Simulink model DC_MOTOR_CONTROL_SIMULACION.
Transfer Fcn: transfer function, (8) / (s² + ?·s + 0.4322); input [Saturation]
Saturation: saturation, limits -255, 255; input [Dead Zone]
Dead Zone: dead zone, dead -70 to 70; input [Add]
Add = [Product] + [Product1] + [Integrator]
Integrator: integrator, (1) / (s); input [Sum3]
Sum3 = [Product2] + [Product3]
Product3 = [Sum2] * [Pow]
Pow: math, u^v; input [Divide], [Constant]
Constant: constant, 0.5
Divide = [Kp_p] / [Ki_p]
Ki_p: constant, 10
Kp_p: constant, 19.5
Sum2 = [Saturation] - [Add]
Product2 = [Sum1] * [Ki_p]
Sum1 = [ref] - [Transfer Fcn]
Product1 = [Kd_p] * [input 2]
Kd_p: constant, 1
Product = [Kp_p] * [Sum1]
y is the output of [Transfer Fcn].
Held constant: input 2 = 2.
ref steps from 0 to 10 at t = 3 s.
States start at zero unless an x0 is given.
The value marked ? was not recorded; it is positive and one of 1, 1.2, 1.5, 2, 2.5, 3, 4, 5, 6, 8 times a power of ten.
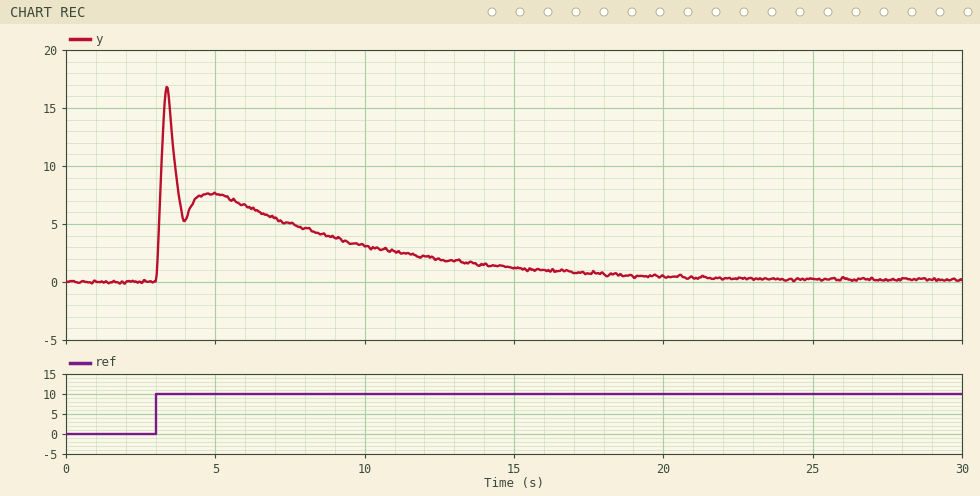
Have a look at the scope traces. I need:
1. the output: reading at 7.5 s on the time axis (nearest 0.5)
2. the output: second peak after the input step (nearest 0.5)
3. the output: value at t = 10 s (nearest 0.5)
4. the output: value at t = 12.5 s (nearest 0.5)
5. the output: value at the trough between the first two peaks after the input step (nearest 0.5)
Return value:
5.0
7.5
3.0
2.0
5.5
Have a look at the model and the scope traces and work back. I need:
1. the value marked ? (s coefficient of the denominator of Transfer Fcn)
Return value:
2.5
